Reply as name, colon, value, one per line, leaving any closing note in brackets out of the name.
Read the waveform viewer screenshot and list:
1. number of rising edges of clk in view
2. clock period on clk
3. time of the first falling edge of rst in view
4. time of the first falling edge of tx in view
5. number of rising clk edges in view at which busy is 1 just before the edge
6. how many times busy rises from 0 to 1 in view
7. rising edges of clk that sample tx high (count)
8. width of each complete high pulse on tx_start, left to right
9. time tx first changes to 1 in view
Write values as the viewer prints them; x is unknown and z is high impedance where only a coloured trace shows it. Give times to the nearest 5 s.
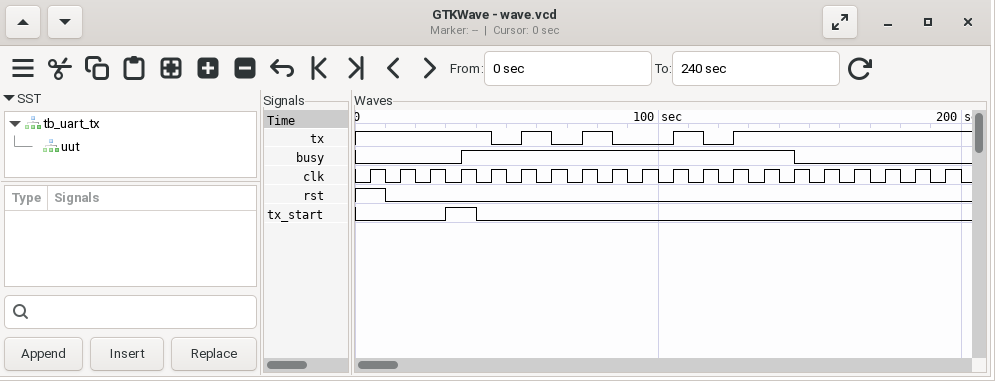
number of rising edges of clk in view: 20
clock period on clk: 10 s
time of the first falling edge of rst in view: 10 s
time of the first falling edge of tx in view: 45 s
number of rising clk edges in view at which busy is 1 just before the edge: 11
how many times busy rises from 0 to 1 in view: 1
rising edges of clk that sample tx high: 15
width of each complete high pulse on tx_start, left to right: 10 s
time tx first changes to 1 in view: 55 s
